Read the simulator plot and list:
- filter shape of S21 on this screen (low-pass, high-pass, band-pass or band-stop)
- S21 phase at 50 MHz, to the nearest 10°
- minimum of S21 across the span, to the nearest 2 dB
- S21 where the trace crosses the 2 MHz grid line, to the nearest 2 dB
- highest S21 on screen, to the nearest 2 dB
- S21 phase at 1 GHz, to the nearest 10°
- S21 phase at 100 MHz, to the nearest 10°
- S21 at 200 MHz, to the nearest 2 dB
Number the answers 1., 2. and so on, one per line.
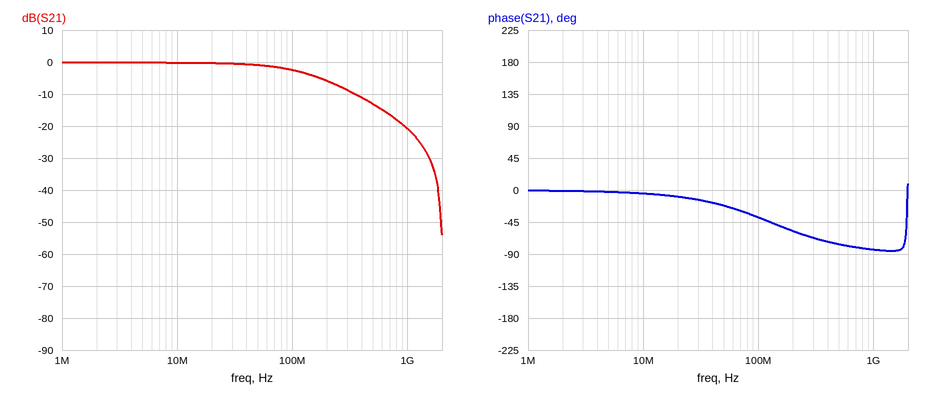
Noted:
1. low-pass
2. -20°
3. -54 dB
4. 0 dB
5. 0 dB
6. -80°
7. -40°
8. -6 dB
